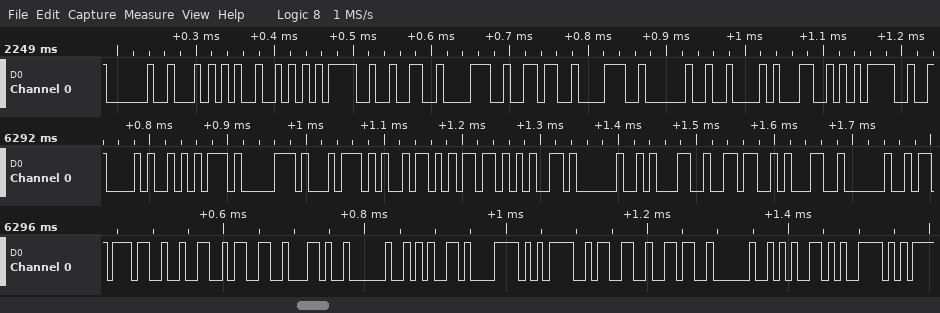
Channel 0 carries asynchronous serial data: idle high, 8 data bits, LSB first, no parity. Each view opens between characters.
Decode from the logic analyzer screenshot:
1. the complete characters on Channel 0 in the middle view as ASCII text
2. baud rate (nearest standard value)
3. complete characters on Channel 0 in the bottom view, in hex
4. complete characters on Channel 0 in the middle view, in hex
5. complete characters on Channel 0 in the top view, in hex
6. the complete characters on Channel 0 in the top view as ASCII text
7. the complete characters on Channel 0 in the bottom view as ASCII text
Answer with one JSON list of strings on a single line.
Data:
["\"(uptime 161 \"", "115200 baud", "37, 32, 33, 2C, 20, 65, 78, 3D, 33, 36, 20, 65, 79", "28, 75, 70, 74, 69, 6D, 65, 20, 31, 36, 31, 20", "20, 54, 52, 3D, 32, 38, 36, 38, 20, 42, 4C, 3D", "\" TR=2868 BL=\"", "\"723, ex=36 ey\""]
